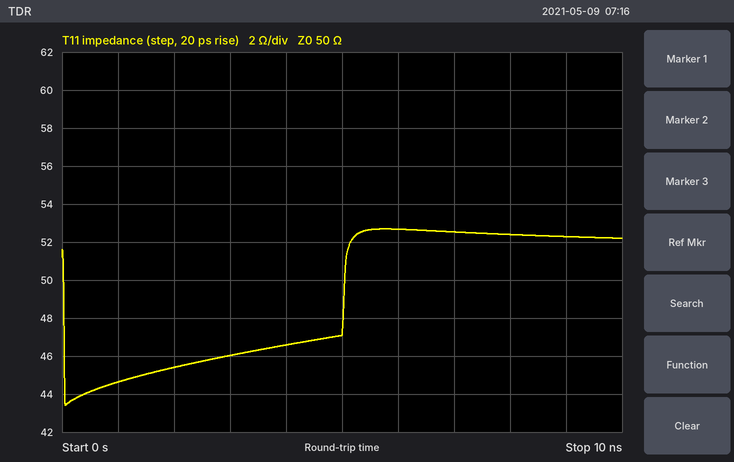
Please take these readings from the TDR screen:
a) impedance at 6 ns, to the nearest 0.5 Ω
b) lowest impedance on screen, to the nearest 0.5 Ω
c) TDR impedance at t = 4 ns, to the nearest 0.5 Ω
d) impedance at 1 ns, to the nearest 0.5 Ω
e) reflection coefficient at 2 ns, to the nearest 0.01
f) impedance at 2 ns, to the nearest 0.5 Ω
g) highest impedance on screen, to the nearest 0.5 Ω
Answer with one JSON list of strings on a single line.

["52.5 Ω", "43.5 Ω", "46.5 Ω", "44.5 Ω", "-0.05", "45.5 Ω", "52.5 Ω"]
